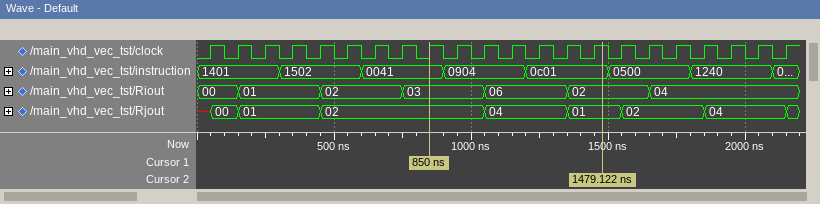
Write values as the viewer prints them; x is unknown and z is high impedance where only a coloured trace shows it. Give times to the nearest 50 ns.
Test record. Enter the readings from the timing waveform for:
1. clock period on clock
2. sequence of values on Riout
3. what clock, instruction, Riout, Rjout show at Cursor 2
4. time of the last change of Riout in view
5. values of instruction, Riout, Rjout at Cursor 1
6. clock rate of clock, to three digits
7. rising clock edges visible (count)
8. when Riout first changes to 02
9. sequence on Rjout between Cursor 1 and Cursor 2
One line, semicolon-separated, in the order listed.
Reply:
100 ns; 00, 01, 02, 03, 06, 02, 04; clock=1, instruction=0c01, Riout=02, Rjout=01; 1650 ns; instruction=0041, Riout=03, Rjout=02; 10.0 MHz; 22; 450 ns; 02, 04, 01
